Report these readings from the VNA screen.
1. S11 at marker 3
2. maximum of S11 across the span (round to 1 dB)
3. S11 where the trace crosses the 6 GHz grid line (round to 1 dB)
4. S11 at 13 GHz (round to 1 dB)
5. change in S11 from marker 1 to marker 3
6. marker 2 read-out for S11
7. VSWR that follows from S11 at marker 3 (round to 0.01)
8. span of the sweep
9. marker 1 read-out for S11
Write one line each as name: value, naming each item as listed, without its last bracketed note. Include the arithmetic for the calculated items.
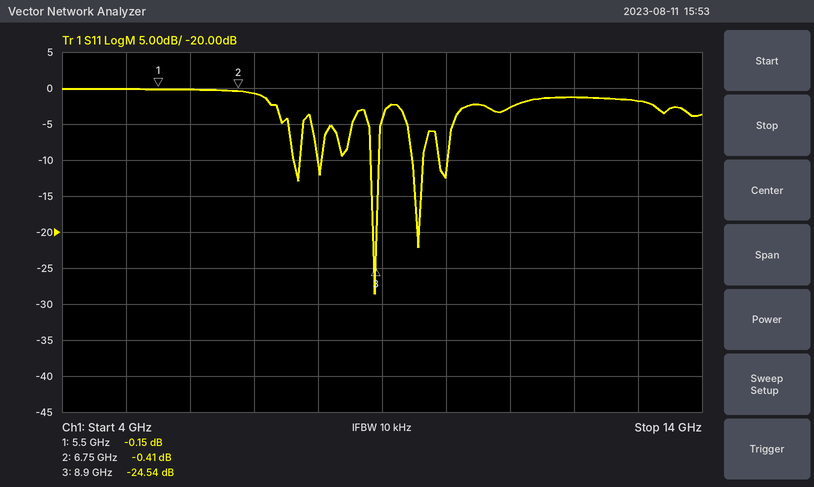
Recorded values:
S11 at marker 3: -24.54 dB
maximum of S11 across the span: 0 dB
S11 where the trace crosses the 6 GHz grid line: 0 dB
S11 at 13 GHz: -2 dB
change in S11 from marker 1 to marker 3: -24.54 − (-0.15) = -24.39 dB
marker 2 read-out for S11: -0.41 dB
VSWR that follows from S11 at marker 3: (1 + 0.0593)/(1 − 0.0593) ≈ 1.13
span of the sweep: 10 GHz
marker 1 read-out for S11: -0.15 dB
